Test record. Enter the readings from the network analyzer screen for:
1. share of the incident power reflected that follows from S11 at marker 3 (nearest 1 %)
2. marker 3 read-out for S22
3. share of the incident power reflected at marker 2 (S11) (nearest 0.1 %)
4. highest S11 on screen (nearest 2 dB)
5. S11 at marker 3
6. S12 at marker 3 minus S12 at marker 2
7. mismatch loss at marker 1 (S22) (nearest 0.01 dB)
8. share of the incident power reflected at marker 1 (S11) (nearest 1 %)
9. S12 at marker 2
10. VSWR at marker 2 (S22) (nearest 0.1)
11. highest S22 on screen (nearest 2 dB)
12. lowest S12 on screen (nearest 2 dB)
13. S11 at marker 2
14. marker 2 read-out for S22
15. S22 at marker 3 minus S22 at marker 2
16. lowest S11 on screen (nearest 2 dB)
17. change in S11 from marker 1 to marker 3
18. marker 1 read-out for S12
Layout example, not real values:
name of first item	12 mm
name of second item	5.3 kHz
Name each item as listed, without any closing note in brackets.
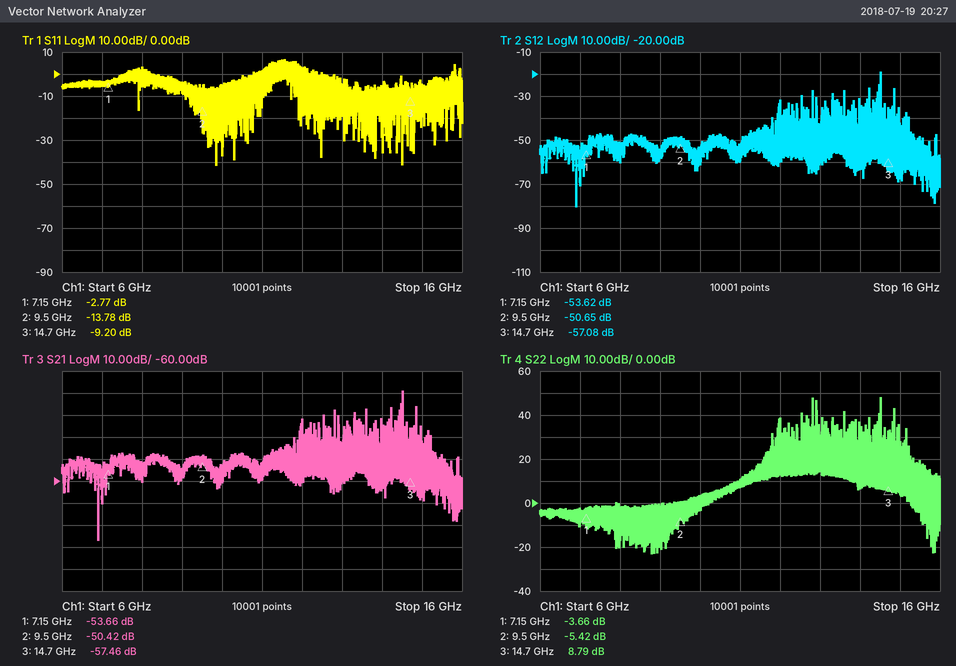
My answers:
share of the incident power reflected that follows from S11 at marker 3	12 %
marker 3 read-out for S22	8.79 dB
share of the incident power reflected at marker 2 (S11)	4.2 %
highest S11 on screen	6 dB
S11 at marker 3	-9.20 dB
S12 at marker 3 minus S12 at marker 2	-6.43 dB
mismatch loss at marker 1 (S22)	2.45 dB
share of the incident power reflected at marker 1 (S11)	53 %
S12 at marker 2	-50.65 dB
VSWR at marker 2 (S22)	3.3
highest S22 on screen	48 dB
lowest S12 on screen	-80 dB
S11 at marker 2	-13.78 dB
marker 2 read-out for S22	-5.42 dB
S22 at marker 3 minus S22 at marker 2	14.21 dB
lowest S11 on screen	-42 dB
change in S11 from marker 1 to marker 3	-6.43 dB
marker 1 read-out for S12	-53.62 dB
